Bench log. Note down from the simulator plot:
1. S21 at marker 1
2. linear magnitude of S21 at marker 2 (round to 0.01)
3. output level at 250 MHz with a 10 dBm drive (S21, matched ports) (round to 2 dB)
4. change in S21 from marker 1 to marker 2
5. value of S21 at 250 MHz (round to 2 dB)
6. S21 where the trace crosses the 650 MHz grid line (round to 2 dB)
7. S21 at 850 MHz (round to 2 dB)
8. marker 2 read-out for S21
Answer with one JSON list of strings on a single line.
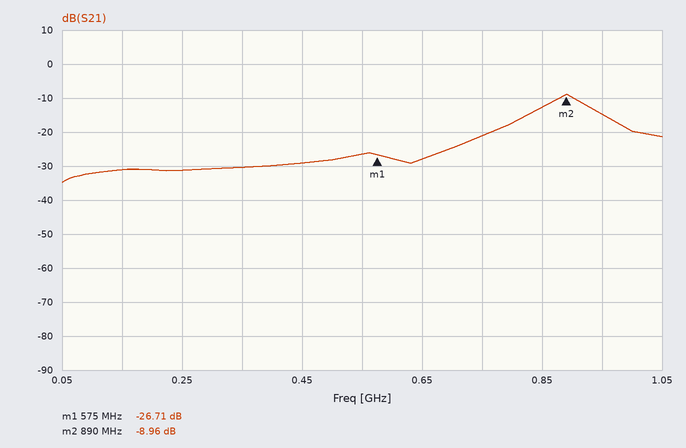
["-26.71 dB", "0.36", "-22 dBm", "17.75 dB", "-32 dB", "-28 dB", "-12 dB", "-8.96 dB"]
